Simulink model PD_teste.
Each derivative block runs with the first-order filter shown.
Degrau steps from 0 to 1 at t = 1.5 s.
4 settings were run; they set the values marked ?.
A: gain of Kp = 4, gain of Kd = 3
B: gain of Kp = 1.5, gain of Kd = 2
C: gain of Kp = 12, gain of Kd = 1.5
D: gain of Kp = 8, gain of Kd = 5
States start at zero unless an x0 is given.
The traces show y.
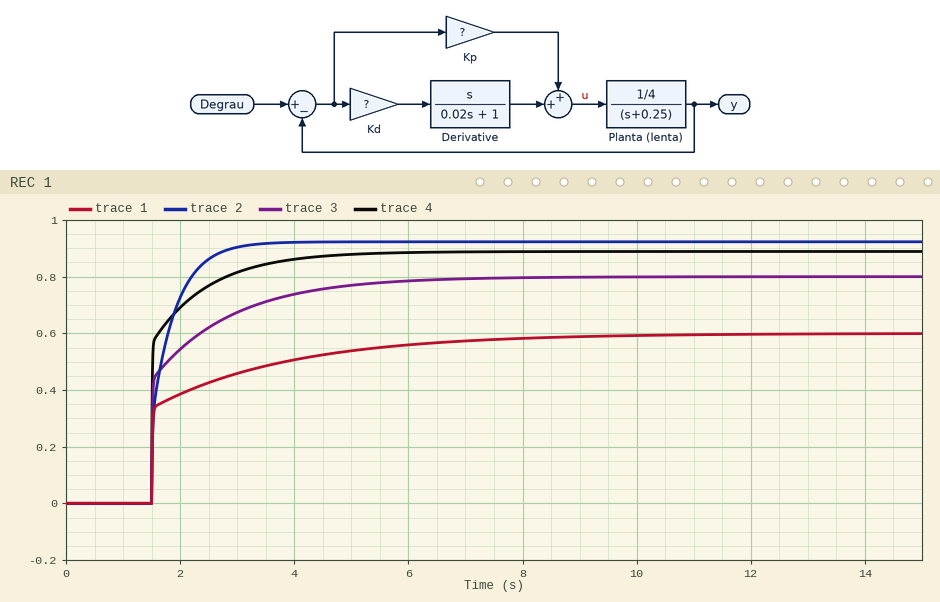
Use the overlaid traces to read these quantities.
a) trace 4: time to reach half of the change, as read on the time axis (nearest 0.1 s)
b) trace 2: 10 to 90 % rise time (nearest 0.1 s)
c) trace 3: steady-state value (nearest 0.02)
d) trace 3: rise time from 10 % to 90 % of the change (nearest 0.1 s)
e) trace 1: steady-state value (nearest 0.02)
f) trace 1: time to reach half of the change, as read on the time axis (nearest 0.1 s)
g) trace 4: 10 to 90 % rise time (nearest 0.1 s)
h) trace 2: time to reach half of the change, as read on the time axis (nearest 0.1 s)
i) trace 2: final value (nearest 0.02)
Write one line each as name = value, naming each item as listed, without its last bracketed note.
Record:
trace 4: time to reach half of the change, as read on the time axis = 1.5 s
trace 2: 10 to 90 % rise time = 0.8 s
trace 3: steady-state value = 0.80
trace 3: rise time from 10 % to 90 % of the change = 2.1 s
trace 1: steady-state value = 0.60
trace 1: time to reach half of the change, as read on the time axis = 1.5 s
trace 4: 10 to 90 % rise time = 1.3 s
trace 2: time to reach half of the change, as read on the time axis = 1.6 s
trace 2: final value = 0.92
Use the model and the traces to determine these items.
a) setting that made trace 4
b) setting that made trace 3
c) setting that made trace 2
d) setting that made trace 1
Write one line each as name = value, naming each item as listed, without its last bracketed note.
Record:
setting that made trace 4 = D
setting that made trace 3 = A
setting that made trace 2 = C
setting that made trace 1 = B
